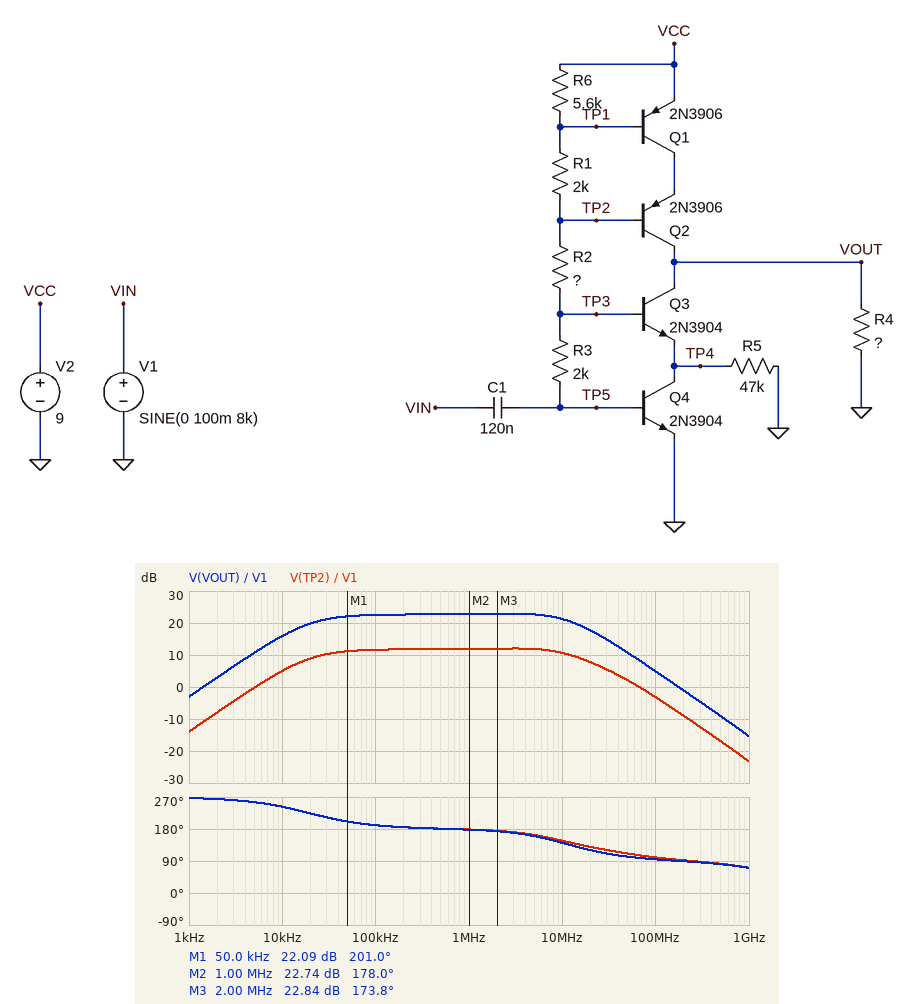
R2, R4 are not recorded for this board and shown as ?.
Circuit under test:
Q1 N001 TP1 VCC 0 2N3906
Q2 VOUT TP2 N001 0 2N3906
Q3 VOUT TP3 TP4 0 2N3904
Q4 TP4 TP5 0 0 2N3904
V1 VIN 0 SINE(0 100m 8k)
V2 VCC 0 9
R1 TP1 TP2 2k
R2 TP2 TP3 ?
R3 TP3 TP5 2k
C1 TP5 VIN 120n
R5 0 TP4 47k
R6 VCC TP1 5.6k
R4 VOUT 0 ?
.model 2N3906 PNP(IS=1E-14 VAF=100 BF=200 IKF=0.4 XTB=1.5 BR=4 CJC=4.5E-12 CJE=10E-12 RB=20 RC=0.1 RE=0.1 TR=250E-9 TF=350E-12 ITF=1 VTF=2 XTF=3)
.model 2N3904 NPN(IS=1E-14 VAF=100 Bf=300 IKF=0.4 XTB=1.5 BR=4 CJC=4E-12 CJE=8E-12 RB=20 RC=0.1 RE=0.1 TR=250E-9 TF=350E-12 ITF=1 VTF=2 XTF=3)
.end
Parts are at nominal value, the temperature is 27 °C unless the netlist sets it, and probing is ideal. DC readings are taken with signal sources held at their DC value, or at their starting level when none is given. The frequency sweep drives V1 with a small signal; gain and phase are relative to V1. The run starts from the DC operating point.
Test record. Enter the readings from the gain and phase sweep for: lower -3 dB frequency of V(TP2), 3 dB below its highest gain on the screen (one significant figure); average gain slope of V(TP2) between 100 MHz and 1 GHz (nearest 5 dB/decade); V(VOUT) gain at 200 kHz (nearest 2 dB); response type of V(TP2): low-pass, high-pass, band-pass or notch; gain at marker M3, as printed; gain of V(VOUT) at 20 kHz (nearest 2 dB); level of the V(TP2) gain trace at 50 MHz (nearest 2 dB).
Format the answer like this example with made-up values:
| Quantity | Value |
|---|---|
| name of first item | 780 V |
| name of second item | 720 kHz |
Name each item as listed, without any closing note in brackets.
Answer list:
| Quantity | Value |
|---|---|
| lower -3 dB frequency of V(TP2), 3 dB below its highest gain on the screen | 20 kHz |
| average gain slope of V(TP2) between 100 MHz and 1 GHz | -20 dB/decade |
| V(VOUT) gain at 200 kHz | 22 dB |
| response type of V(TP2): low-pass, high-pass, band-pass or notch | band-pass |
| gain at marker M3, as printed | 22.84 dB |
| gain of V(VOUT) at 20 kHz | 20 dB |
| level of the V(TP2) gain trace at 50 MHz | 2 dB |
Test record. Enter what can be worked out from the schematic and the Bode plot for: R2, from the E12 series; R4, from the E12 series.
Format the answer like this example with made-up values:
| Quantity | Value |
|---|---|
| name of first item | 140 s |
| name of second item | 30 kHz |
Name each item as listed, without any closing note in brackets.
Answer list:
| Quantity | Value |
|---|---|
| R2, from the E12 series | 2.7 kΩ |
| R4, from the E12 series | 10 Ω |
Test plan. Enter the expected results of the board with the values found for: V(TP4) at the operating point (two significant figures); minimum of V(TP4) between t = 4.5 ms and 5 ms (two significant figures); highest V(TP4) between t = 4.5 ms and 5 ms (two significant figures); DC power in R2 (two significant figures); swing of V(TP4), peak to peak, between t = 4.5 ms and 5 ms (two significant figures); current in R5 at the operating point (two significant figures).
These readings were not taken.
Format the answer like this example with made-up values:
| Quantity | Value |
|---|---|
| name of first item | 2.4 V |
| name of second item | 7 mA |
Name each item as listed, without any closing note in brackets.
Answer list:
| Quantity | Value |
|---|---|
| V(TP4) at the operating point | 520 mV |
| minimum of V(TP4) between t = 4.5 ms and 5 ms | 160 mV |
| highest V(TP4) between t = 4.5 ms and 5 ms | 1.0 V |
| DC power in R2 | 8.7 mW |
| swing of V(TP4), peak to peak, between t = 4.5 ms and 5 ms | 880 mV |
| current in R5 at the operating point | 11 µA |
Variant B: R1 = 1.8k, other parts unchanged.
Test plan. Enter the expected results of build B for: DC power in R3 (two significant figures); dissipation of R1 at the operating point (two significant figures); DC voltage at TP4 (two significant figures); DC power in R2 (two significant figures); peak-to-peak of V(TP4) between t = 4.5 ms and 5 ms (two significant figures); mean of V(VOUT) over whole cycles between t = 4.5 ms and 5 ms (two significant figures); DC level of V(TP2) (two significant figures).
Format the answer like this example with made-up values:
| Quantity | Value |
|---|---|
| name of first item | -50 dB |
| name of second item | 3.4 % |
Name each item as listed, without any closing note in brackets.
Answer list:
| Quantity | Value |
|---|---|
| DC power in R3 | 160 µW |
| dissipation of R1 at the operating point | 1.9 mW |
| DC voltage at TP4 | 540 mV |
| DC power in R2 | 9.2 mW |
| peak-to-peak of V(TP4) between t = 4.5 ms and 5 ms | 890 mV |
| mean of V(VOUT) over whole cycles between t = 4.5 ms and 5 ms | 670 mV |
| DC level of V(TP2) | 6.3 V |
